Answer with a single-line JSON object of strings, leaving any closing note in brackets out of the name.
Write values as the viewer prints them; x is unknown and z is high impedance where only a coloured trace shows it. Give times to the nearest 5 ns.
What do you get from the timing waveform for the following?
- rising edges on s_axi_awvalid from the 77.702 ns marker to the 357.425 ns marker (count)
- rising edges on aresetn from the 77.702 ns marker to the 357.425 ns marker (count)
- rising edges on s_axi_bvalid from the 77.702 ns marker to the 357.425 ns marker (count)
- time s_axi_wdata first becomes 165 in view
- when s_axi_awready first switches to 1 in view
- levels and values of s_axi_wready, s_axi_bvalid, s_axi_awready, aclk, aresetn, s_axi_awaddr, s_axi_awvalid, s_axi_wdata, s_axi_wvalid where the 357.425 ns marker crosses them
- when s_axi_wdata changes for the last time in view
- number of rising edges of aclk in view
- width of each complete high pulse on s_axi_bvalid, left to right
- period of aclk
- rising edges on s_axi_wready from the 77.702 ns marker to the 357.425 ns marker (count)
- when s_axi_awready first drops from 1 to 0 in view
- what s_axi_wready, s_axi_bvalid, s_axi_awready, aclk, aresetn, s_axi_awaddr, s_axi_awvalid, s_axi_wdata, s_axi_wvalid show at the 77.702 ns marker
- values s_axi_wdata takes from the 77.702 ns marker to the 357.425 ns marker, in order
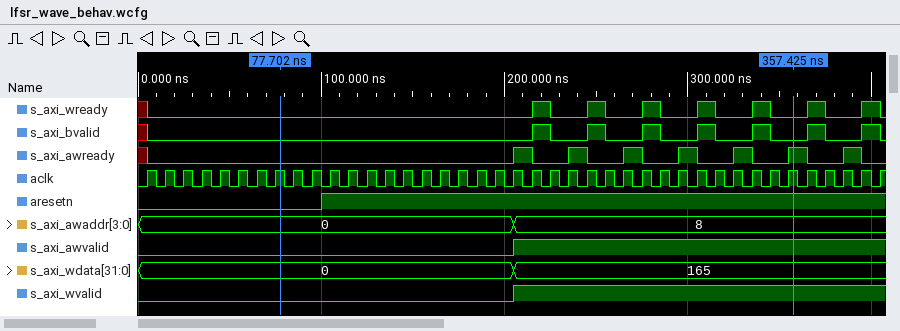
{"rising edges on s_axi_awvalid from the 77.702 ns marker to the 357.425 ns marker": "1", "rising edges on aresetn from the 77.702 ns marker to the 357.425 ns marker": "1", "rising edges on s_axi_bvalid from the 77.702 ns marker to the 357.425 ns marker": "5", "time s_axi_wdata first becomes 165 in view": "205 ns", "when s_axi_awready first switches to 1 in view": "205 ns", "levels and values of s_axi_wready, s_axi_bvalid, s_axi_awready, aclk, aresetn, s_axi_awaddr, s_axi_awvalid, s_axi_wdata, s_axi_wvalid where the 357.425 ns marker crosses them": "s_axi_wready=0, s_axi_bvalid=0, s_axi_awready=1, aclk=1, aresetn=1, s_axi_awaddr=8, s_axi_awvalid=1, s_axi_wdata=165, s_axi_wvalid=1", "when s_axi_wdata changes for the last time in view": "205 ns", "number of rising edges of aclk in view": "41", "width of each complete high pulse on s_axi_bvalid, left to right": "10 ns, 10 ns, 10 ns, 10 ns, 10 ns, 10 ns, 10 ns", "period of aclk": "10 ns", "rising edges on s_axi_wready from the 77.702 ns marker to the 357.425 ns marker": "5", "when s_axi_awready first drops from 1 to 0 in view": "215 ns", "what s_axi_wready, s_axi_bvalid, s_axi_awready, aclk, aresetn, s_axi_awaddr, s_axi_awvalid, s_axi_wdata, s_axi_wvalid show at the 77.702 ns marker": "s_axi_wready=0, s_axi_bvalid=0, s_axi_awready=0, aclk=1, aresetn=0, s_axi_awaddr=0, s_axi_awvalid=0, s_axi_wdata=0, s_axi_wvalid=0", "values s_axi_wdata takes from the 77.702 ns marker to the 357.425 ns marker, in order": "0, 165"}
